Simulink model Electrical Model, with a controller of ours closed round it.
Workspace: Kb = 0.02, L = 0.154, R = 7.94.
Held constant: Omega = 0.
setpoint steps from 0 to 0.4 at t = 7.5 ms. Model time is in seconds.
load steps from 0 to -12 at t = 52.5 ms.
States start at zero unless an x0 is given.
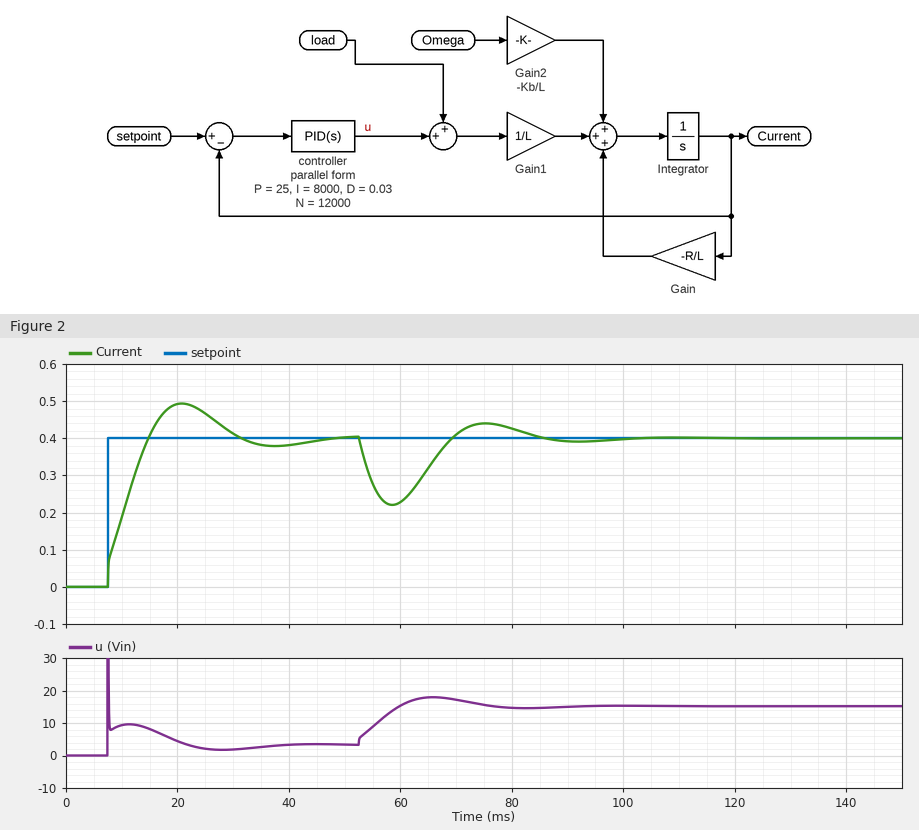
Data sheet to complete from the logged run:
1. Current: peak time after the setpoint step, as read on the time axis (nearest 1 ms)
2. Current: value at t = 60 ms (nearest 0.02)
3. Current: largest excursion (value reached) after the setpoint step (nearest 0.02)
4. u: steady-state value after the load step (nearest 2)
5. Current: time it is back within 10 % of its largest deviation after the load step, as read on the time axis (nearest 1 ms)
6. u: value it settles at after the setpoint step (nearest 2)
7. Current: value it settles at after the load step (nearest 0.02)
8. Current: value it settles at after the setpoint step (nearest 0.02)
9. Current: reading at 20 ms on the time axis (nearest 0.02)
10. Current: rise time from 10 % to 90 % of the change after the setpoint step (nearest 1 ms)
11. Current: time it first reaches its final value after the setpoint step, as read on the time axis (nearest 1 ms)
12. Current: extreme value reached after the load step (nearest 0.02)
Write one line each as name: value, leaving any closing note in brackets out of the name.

Current: peak time after the setpoint step, as read on the time axis: 21 ms
Current: value at t = 60 ms: 0.22
Current: largest excursion (value reached) after the setpoint step: 0.50
u: steady-state value after the load step: 16
Current: time it is back within 10 % of its largest deviation after the load step, as read on the time axis: 82 ms
u: value it settles at after the setpoint step: 4
Current: value it settles at after the load step: 0.40
Current: value it settles at after the setpoint step: 0.40
Current: reading at 20 ms on the time axis: 0.50
Current: rise time from 10 % to 90 % of the change after the setpoint step: 6 ms
Current: time it first reaches its final value after the setpoint step, as read on the time axis: 15 ms
Current: extreme value reached after the load step: 0.22
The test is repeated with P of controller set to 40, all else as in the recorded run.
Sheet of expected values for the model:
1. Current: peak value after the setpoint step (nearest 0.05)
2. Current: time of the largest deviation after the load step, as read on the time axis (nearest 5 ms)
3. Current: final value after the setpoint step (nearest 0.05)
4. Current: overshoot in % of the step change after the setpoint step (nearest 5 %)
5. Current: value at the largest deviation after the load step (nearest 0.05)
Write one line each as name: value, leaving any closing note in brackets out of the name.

Current: peak value after the setpoint step: 0.45
Current: time of the largest deviation after the load step, as read on the time axis: 60 ms
Current: final value after the setpoint step: 0.40
Current: overshoot in % of the step change after the setpoint step: 15 %
Current: value at the largest deviation after the load step: 0.25
